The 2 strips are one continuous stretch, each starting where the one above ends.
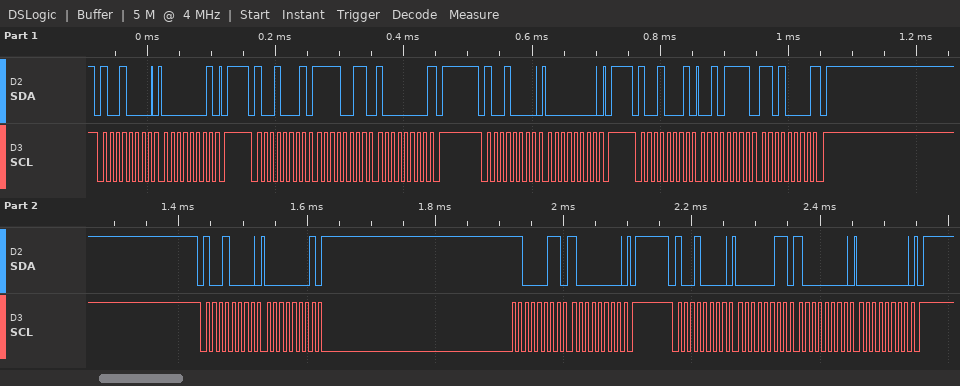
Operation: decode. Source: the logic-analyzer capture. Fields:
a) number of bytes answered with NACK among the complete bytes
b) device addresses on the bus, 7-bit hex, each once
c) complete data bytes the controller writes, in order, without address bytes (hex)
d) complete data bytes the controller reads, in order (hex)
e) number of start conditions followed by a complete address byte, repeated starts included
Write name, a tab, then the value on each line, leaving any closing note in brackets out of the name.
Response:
number of bytes answered with NACK among the complete bytes	2
device addresses on the bus, 7-bit hex, each once	0x48
complete data bytes the controller writes, in order, without address bytes	01 00 01 C3 80 03 80 00
complete data bytes the controller reads, in order	F3 80 2F D0
number of start conditions followed by a complete address byte, repeated starts included	6
